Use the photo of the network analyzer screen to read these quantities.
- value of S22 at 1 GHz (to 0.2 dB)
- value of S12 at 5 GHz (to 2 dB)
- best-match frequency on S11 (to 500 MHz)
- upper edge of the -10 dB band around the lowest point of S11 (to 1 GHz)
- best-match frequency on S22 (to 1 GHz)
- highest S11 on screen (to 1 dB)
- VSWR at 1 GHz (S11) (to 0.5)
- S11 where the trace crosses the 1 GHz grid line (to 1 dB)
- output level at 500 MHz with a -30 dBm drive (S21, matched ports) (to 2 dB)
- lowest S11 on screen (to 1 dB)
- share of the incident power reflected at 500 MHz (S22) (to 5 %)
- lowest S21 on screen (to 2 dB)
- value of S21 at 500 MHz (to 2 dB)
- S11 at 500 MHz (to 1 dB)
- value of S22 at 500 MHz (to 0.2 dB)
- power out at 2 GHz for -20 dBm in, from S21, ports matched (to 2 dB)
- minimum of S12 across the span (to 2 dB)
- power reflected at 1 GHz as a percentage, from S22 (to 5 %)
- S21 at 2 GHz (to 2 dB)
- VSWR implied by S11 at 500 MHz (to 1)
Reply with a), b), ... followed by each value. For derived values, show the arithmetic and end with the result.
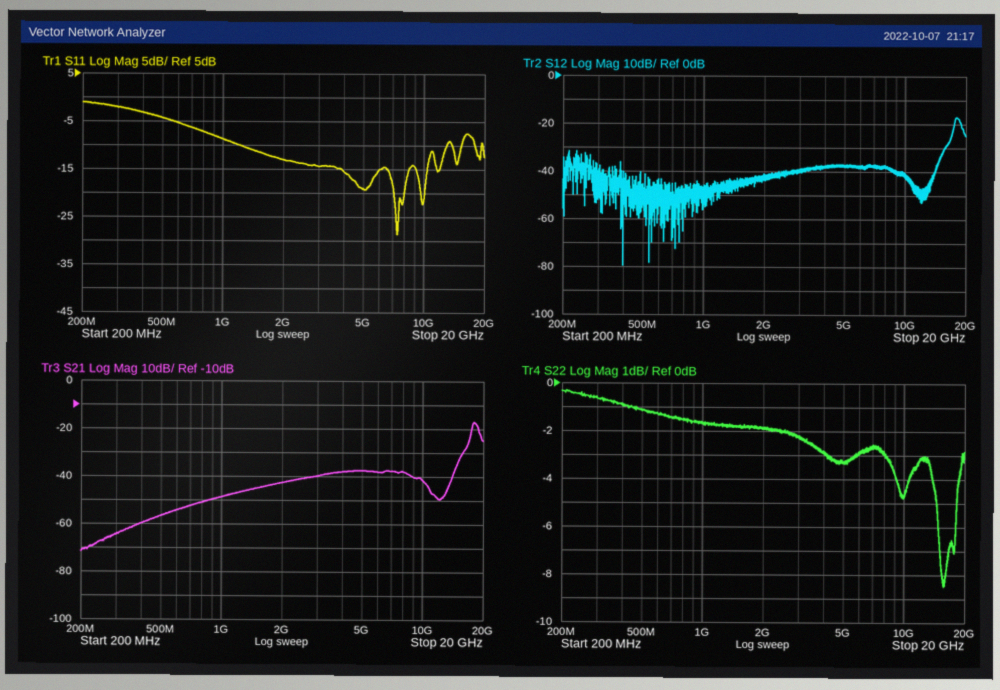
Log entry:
a) -1.6 dB
b) -38 dB
c) 7.5 GHz
d) 13 GHz
e) 16 GHz
f) -1 dB
g) |Γ| = 10^(-9/20) = 0.3548; VSWR = (1 + 0.3548)/(1 − 0.3548) ≈ 2.10, so 2.0 to the nearest 0.5
h) -9 dB
i) -30 dBm + (-56 dB) = -86 dBm
j) -29 dB
k) 10^(-1.2/10) ≈ 75.9 %, so 75 % to the nearest 5 %
l) -72 dB
m) -56 dB
n) -4 dB
o) -1.2 dB
p) -20 dBm + (-42 dB) = -62 dBm
q) -80 dB
r) 10^(-1.6/10) ≈ 69.2 %, so 70 % to the nearest 5 %
s) -42 dB
t) |Γ| = 10^(-4/20) = 0.6310; VSWR = (1 + 0.6310)/(1 − 0.6310) ≈ 4
